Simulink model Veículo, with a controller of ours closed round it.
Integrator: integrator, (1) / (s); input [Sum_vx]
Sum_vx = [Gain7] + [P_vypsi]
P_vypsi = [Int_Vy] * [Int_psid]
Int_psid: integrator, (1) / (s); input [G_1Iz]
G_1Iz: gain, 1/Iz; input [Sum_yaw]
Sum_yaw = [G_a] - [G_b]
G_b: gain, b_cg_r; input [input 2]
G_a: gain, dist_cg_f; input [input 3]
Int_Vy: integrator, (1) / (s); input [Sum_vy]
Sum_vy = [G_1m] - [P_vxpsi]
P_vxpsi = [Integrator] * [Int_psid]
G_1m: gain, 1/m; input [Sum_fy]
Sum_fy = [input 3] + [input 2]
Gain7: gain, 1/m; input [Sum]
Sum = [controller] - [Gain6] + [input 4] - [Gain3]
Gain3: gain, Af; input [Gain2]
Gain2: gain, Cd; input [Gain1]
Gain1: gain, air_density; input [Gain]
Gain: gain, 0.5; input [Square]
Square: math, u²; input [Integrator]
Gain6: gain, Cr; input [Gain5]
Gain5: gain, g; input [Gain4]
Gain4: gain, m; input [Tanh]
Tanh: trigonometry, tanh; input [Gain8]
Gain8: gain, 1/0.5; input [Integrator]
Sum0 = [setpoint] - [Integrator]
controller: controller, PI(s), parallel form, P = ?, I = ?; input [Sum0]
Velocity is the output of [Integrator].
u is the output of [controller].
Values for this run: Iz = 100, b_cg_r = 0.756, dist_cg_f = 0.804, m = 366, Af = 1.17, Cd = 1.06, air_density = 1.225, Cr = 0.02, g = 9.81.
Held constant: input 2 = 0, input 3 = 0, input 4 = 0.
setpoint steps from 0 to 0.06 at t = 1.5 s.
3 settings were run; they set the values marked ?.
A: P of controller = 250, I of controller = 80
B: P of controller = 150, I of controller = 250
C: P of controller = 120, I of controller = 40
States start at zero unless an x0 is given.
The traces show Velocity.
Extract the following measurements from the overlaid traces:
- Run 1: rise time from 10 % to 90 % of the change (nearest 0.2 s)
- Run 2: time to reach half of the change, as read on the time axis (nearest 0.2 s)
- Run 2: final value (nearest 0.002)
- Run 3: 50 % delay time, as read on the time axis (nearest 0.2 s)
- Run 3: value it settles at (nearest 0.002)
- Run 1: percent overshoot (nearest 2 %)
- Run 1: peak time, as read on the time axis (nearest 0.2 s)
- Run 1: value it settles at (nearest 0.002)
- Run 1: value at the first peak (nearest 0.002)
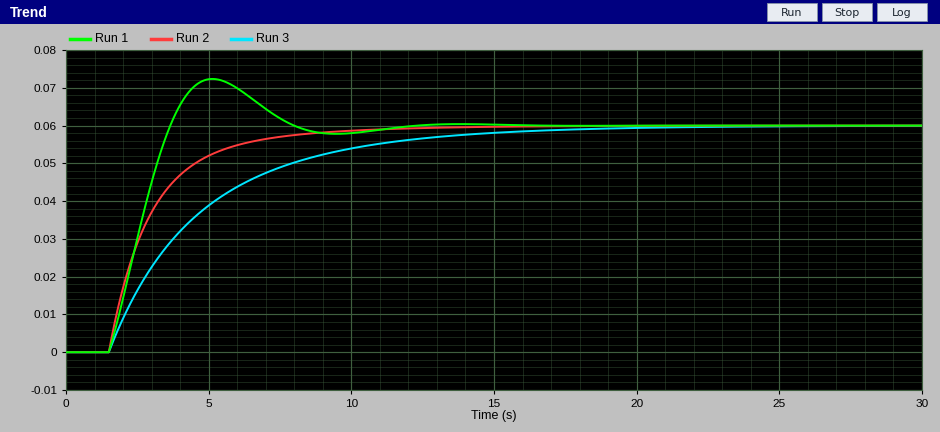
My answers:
1.6 s
2.6 s
0.060
3.8 s
0.060
20 %
5.2 s
0.060
0.072
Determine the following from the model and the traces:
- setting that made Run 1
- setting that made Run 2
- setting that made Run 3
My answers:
B
A
C
